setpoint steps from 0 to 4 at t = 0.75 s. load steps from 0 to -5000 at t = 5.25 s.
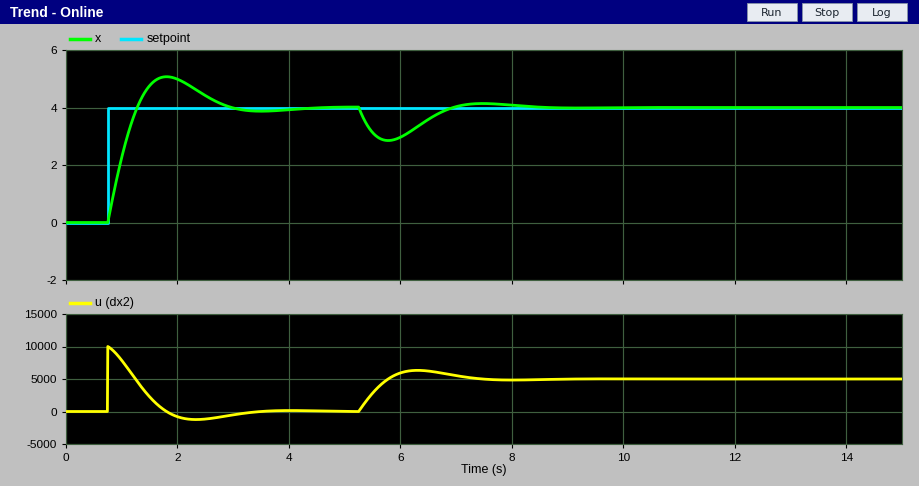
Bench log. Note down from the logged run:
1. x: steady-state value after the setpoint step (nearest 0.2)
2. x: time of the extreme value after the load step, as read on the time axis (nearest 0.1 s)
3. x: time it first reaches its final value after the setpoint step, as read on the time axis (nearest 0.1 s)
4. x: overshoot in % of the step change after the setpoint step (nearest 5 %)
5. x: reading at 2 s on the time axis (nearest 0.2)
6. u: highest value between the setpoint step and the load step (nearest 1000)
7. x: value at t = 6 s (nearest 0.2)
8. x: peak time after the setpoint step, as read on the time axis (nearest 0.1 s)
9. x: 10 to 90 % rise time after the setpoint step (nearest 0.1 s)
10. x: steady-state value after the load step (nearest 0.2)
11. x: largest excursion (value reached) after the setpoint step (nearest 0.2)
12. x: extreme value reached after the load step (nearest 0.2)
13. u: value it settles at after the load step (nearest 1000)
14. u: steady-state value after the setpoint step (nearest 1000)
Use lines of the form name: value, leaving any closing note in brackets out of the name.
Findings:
x: steady-state value after the setpoint step: 4.0
x: time of the extreme value after the load step, as read on the time axis: 5.8 s
x: time it first reaches its final value after the setpoint step, as read on the time axis: 1.3 s
x: overshoot in % of the step change after the setpoint step: 25 %
x: reading at 2 s on the time axis: 5.0
u: highest value between the setpoint step and the load step: 10000
x: value at t = 6 s: 3.0
x: peak time after the setpoint step, as read on the time axis: 1.8 s
x: 10 to 90 % rise time after the setpoint step: 0.4 s
x: steady-state value after the load step: 4.0
x: largest excursion (value reached) after the setpoint step: 5.0
x: extreme value reached after the load step: 2.8
u: value it settles at after the load step: 5000
u: steady-state value after the setpoint step: 0
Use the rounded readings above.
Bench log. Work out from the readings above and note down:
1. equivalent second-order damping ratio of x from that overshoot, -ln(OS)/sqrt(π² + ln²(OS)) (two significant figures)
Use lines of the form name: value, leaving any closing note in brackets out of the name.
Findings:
equivalent second-order damping ratio of x from that overshoot, -ln(OS)/sqrt(π² + ln²(OS)): 0.40
